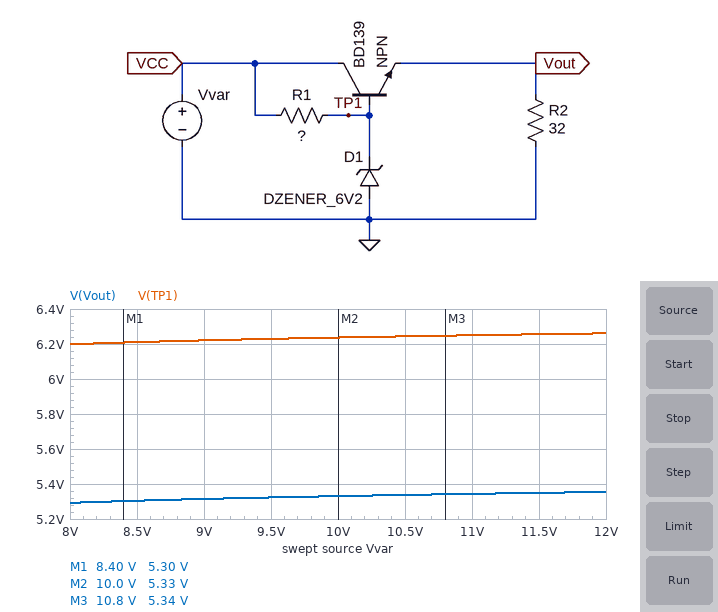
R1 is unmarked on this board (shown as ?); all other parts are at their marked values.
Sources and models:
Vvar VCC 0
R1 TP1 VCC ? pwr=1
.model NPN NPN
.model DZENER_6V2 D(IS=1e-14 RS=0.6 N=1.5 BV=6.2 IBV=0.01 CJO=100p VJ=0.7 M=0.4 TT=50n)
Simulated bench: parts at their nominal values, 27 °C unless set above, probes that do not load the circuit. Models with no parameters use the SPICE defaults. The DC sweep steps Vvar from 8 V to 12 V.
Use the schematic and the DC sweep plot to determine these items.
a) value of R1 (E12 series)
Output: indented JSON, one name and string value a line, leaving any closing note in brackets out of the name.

{
  "value of R1": "180 Ω"
}
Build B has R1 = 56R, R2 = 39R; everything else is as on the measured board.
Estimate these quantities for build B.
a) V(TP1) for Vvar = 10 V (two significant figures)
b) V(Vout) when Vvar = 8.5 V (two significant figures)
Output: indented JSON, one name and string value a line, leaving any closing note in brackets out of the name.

{
  "V(TP1) for Vvar = 10 V": "6.3 V",
  "V(Vout) when Vvar = 8.5 V": "5.4 V"
}
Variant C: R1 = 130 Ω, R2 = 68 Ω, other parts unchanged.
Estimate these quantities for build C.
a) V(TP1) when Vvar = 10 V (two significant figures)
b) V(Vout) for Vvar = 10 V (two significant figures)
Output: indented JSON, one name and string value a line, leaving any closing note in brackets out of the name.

{
  "V(TP1) when Vvar = 10 V": "6.3 V",
  "V(Vout) for Vvar = 10 V": "5.4 V"
}
